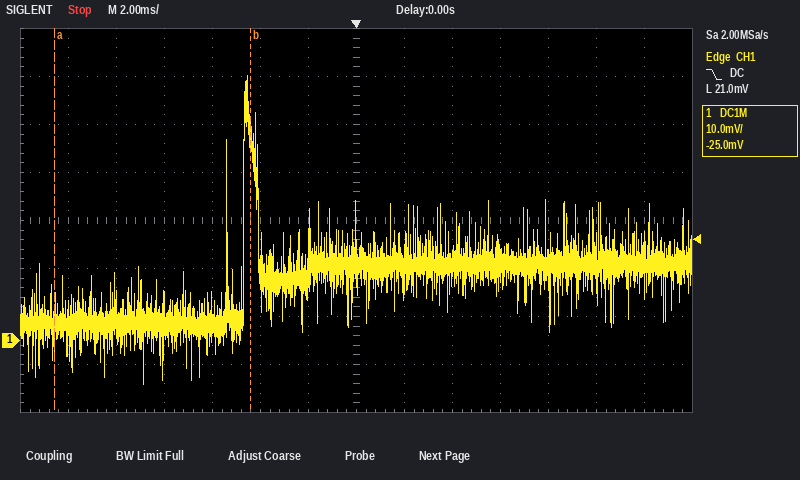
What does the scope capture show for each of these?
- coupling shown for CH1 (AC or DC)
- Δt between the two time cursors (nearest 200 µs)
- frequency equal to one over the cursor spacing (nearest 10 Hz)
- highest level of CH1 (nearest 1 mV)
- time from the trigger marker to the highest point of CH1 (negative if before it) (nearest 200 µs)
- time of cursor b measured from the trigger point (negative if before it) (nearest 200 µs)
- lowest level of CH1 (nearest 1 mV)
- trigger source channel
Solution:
DC
8.2 ms
120 Hz
55 mV
-4.6 ms
-4.4 ms
-9 mV
CH1
